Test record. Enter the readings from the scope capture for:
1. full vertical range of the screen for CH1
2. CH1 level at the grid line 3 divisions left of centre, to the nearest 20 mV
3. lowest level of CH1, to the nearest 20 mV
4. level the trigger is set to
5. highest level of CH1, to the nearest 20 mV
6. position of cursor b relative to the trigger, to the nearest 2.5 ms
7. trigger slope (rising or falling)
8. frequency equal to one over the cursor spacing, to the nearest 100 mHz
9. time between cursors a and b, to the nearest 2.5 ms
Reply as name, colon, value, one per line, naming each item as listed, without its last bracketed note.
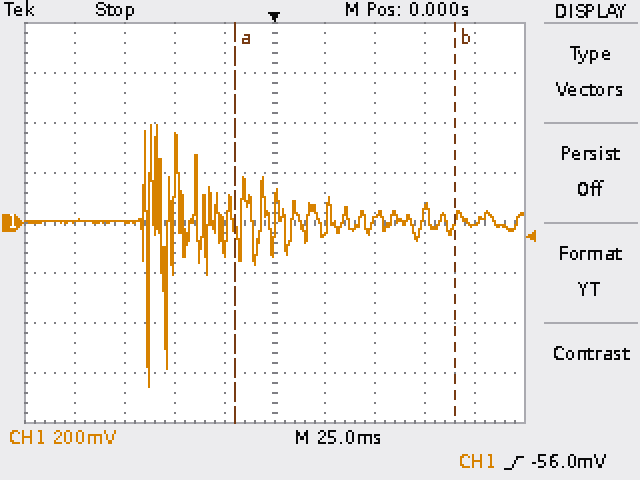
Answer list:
full vertical range of the screen for CH1: 1.6 V
CH1 level at the grid line 3 divisions left of centre, to the nearest 20 mV: 0 mV
lowest level of CH1, to the nearest 20 mV: -660 mV
level the trigger is set to: -56.0 mV
highest level of CH1, to the nearest 20 mV: 400 mV
position of cursor b relative to the trigger, to the nearest 2.5 ms: +90.0 ms
trigger slope: rising
frequency equal to one over the cursor spacing, to the nearest 100 mHz: 9.1 Hz
time between cursors a and b, to the nearest 2.5 ms: 110.0 ms
